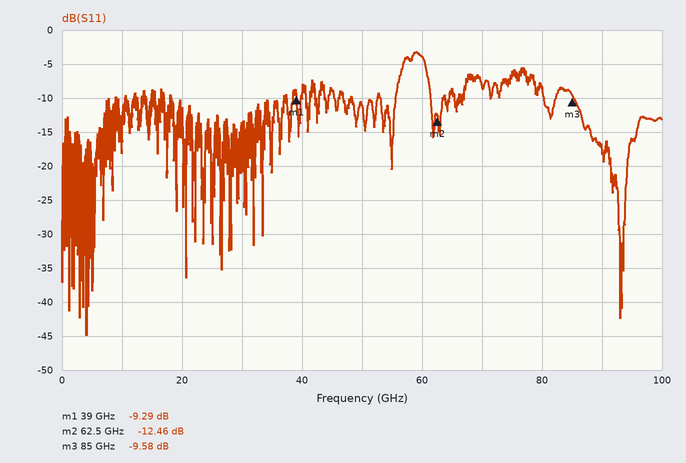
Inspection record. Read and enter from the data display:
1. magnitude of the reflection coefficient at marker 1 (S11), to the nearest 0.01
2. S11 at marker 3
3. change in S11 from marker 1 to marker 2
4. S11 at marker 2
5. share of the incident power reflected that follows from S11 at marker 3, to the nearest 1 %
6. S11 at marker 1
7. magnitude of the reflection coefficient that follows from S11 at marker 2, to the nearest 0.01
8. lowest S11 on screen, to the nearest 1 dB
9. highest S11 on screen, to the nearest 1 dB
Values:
0.34
-9.58 dB
-3.17 dB
-12.46 dB
11 %
-9.29 dB
0.24
-45 dB
-3 dB
